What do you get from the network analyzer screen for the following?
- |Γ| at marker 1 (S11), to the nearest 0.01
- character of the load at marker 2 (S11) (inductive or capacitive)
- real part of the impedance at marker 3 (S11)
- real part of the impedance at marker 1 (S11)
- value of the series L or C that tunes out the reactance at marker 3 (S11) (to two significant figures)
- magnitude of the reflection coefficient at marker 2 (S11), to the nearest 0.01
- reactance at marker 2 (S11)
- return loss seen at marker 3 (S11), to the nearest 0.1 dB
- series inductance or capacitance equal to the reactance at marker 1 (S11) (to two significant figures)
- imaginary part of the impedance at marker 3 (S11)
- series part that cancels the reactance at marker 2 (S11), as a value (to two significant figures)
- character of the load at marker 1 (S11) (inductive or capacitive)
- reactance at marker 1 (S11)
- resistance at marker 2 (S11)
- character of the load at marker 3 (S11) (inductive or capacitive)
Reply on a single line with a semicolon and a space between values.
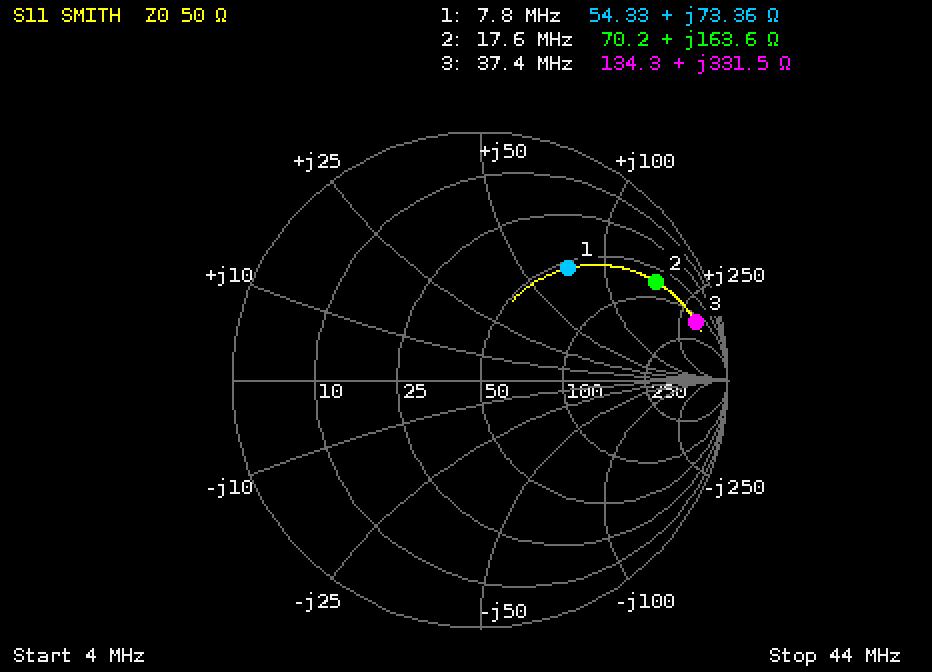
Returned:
0.58; inductive; 134.3 Ω; 54.33 Ω; 13 pF; 0.81; +163.6 Ω; 0.9 dB; 1.5 µH; +331.5 Ω; 55 pF; inductive; +73.36 Ω; 70.2 Ω; inductive
